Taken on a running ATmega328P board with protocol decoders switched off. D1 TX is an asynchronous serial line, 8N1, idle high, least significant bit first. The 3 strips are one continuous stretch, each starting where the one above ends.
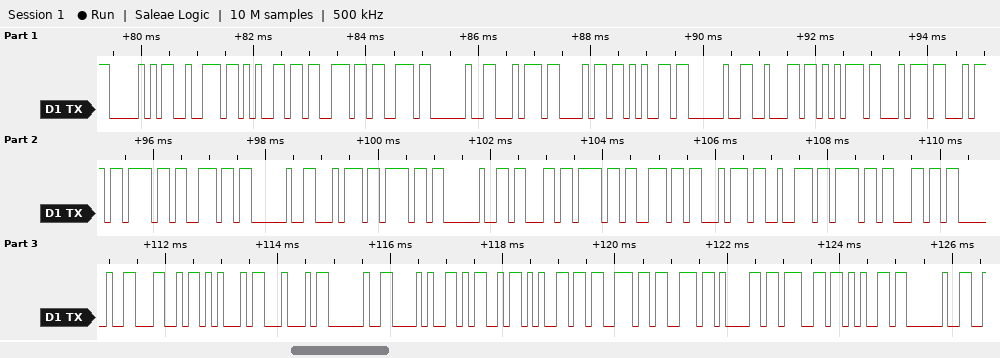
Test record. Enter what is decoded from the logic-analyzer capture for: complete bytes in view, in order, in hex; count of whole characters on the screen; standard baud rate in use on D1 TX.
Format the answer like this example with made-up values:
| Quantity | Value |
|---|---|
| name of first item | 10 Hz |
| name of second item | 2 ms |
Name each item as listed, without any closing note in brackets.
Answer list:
| Quantity | Value |
|---|---|
| complete bytes in view, in order, in hex | 50 72 65 73 73 20 74 68 65 20 62 75 74 74 6F 6E 20 74 6F 20 63 6F 6E 74 72 6F 6C 20 4C 45 44 20 28 4D 65 73 73 61 67 65 20 |
| count of whole characters on the screen | 41 |
| standard baud rate in use on D1 TX | 9600 baud |
